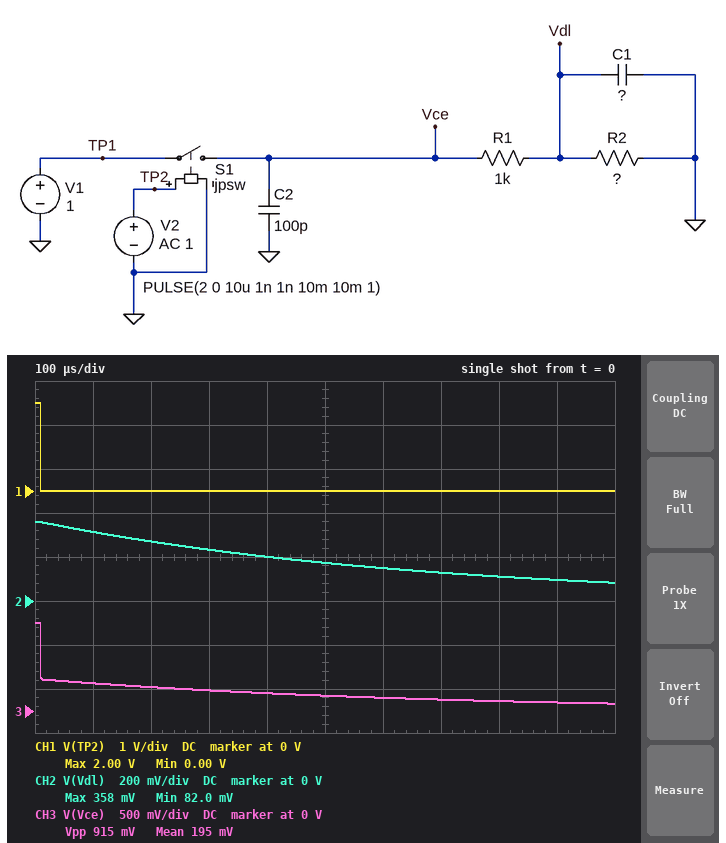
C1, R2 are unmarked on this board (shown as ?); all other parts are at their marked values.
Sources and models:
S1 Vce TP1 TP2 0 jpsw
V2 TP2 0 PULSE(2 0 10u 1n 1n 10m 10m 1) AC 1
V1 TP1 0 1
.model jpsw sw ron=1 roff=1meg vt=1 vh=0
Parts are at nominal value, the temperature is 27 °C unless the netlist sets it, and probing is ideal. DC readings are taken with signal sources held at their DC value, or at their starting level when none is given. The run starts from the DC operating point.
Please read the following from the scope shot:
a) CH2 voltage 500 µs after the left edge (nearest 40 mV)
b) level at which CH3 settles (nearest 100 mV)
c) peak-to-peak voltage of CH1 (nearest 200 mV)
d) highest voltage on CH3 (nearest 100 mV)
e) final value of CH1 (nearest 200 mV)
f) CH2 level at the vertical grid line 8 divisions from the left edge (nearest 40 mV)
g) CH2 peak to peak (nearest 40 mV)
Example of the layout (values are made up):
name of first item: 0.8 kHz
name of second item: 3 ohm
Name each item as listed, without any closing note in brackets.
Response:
CH2 voltage 500 µs after the left edge: 160 mV
level at which CH3 settles: 100 mV
peak-to-peak voltage of CH1: 2.0 V
highest voltage on CH3: 1.0 V
final value of CH1: 0 V
CH2 level at the vertical grid line 8 divisions from the left edge: 120 mV
CH2 peak to peak: 280 mV
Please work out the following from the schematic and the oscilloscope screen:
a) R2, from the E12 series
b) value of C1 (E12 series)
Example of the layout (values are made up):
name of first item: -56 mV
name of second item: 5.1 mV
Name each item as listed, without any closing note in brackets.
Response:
R2, from the E12 series: 560 Ω
value of C1: 1.2 µF
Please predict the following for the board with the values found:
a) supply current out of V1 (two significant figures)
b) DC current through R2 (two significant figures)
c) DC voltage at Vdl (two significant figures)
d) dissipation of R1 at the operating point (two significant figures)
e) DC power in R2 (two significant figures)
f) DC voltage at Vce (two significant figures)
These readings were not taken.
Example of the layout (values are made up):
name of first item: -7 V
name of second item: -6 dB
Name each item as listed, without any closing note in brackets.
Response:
supply current out of V1: 640 µA
DC current through R2: 640 µA
DC voltage at Vdl: 360 mV
dissipation of R1 at the operating point: 410 µW
DC power in R2: 230 µW
DC voltage at Vce: 1.0 V
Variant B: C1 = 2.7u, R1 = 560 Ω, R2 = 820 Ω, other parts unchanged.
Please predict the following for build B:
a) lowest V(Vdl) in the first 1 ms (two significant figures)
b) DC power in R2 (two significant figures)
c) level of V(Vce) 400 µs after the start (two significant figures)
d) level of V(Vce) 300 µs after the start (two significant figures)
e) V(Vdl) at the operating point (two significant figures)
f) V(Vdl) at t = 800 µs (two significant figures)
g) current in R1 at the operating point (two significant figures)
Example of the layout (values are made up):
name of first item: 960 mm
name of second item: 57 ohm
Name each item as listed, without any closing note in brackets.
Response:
lowest V(Vdl) in the first 1 ms: 380 mV
DC power in R2: 430 µW
level of V(Vce) 400 µs after the start: 500 mV
level of V(Vce) 300 µs after the start: 520 mV
V(Vdl) at the operating point: 590 mV
V(Vdl) at t = 800 µs: 420 mV
current in R1 at the operating point: 720 µA
